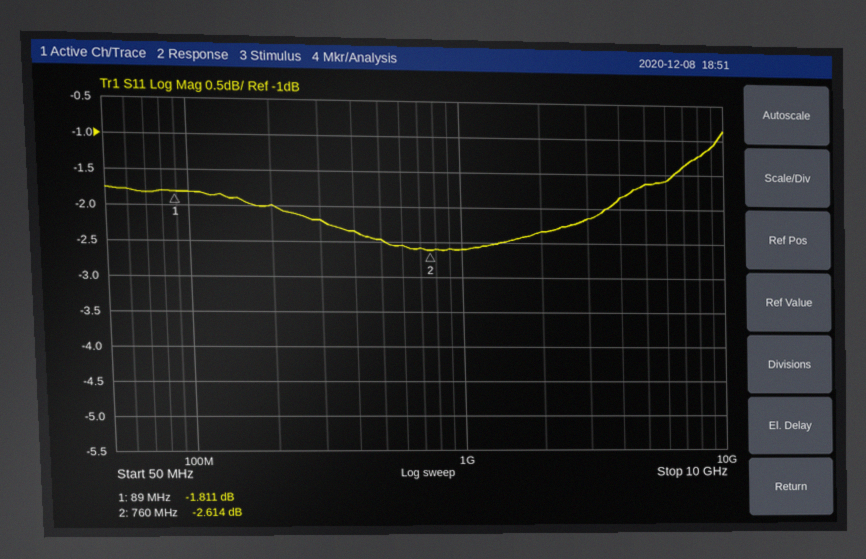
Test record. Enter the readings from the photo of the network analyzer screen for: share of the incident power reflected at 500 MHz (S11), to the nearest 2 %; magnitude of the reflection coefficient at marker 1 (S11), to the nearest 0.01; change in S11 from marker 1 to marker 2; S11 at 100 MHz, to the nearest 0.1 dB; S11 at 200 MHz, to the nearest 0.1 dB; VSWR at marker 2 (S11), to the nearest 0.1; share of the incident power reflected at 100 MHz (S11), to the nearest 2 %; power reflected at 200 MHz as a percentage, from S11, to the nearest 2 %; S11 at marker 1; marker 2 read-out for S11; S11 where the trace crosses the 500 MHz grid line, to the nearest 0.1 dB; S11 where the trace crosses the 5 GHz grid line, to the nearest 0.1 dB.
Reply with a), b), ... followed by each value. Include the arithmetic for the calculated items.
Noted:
a) 10^(-2.5/10) ≈ 56 %
b) 10^(-1.811/20) ≈ 0.81
c) -2.614 − (-1.811) = -0.803 dB
d) -1.8 dB
e) -2.0 dB
f) (1 + 0.7401)/(1 − 0.7401) ≈ 6.7
g) 10^(-1.8/10) ≈ 66 %
h) 10^(-2/10) ≈ 63.1 %, so 64 % to the nearest 2 %
i) -1.811 dB
j) -2.614 dB
k) -2.5 dB
l) -1.6 dB
